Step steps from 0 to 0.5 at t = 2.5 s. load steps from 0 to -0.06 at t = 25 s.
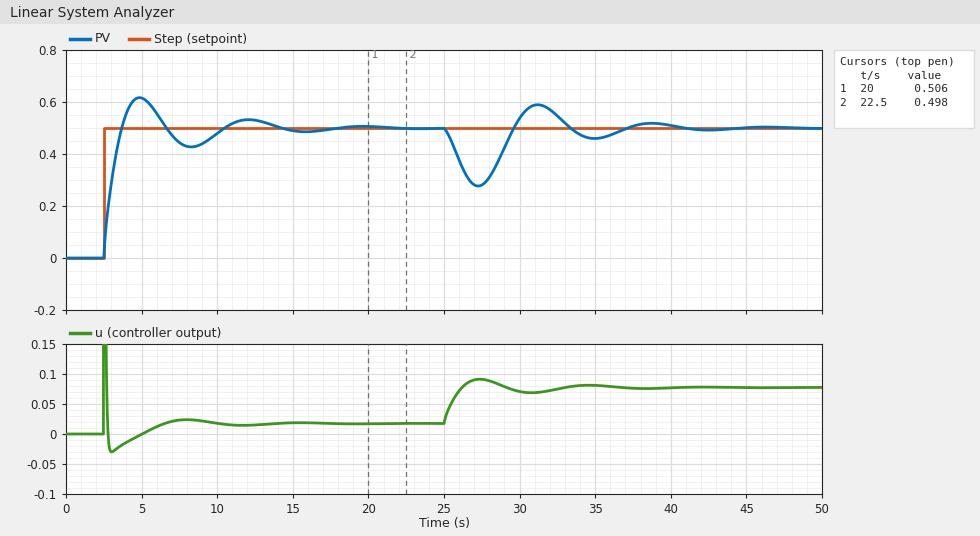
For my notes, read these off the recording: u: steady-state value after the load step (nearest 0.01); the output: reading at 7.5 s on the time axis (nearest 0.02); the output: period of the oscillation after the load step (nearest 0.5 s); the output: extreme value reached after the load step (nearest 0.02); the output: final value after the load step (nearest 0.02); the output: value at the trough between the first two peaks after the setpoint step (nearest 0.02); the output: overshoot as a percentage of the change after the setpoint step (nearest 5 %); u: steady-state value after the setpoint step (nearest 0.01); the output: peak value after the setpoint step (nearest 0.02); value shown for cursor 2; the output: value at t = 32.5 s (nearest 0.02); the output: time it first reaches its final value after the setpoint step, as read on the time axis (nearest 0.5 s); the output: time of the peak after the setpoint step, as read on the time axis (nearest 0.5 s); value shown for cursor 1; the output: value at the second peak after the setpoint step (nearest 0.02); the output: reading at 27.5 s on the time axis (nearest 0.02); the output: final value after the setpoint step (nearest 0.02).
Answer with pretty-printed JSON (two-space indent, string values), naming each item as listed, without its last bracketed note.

{
  "u: steady-state value after the load step": "0.08",
  "the output: reading at 7.5 s on the time axis": "0.44",
  "the output: period of the oscillation after the load step": "7.5 s",
  "the output: extreme value reached after the load step": "0.28",
  "the output: final value after the load step": "0.50",
  "the output: value at the trough between the first two peaks after the setpoint step": "0.42",
  "the output: overshoot as a percentage of the change after the setpoint step": "25 %",
  "u: steady-state value after the setpoint step": "0.02",
  "the output: peak value after the setpoint step": "0.62",
  "value shown for cursor 2": "0.498",
  "the output: value at t = 32.5 s": "0.54",
  "the output: time it first reaches its final value after the setpoint step, as read on the time axis": "3.5 s",
  "the output: time of the peak after the setpoint step, as read on the time axis": "5.0 s",
  "value shown for cursor 1": "0.506",
  "the output: value at the second peak after the setpoint step": "0.54",
  "the output: reading at 27.5 s on the time axis": "0.28",
  "the output: final value after the setpoint step": "0.50"
}
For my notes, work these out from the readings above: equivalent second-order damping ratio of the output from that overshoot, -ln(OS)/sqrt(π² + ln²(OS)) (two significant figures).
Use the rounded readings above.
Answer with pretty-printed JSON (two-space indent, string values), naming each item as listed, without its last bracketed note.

{
  "equivalent second-order damping ratio of the output from that overshoot, -ln(OS)/sqrt(π² + ln²(OS))": "0.40"
}
